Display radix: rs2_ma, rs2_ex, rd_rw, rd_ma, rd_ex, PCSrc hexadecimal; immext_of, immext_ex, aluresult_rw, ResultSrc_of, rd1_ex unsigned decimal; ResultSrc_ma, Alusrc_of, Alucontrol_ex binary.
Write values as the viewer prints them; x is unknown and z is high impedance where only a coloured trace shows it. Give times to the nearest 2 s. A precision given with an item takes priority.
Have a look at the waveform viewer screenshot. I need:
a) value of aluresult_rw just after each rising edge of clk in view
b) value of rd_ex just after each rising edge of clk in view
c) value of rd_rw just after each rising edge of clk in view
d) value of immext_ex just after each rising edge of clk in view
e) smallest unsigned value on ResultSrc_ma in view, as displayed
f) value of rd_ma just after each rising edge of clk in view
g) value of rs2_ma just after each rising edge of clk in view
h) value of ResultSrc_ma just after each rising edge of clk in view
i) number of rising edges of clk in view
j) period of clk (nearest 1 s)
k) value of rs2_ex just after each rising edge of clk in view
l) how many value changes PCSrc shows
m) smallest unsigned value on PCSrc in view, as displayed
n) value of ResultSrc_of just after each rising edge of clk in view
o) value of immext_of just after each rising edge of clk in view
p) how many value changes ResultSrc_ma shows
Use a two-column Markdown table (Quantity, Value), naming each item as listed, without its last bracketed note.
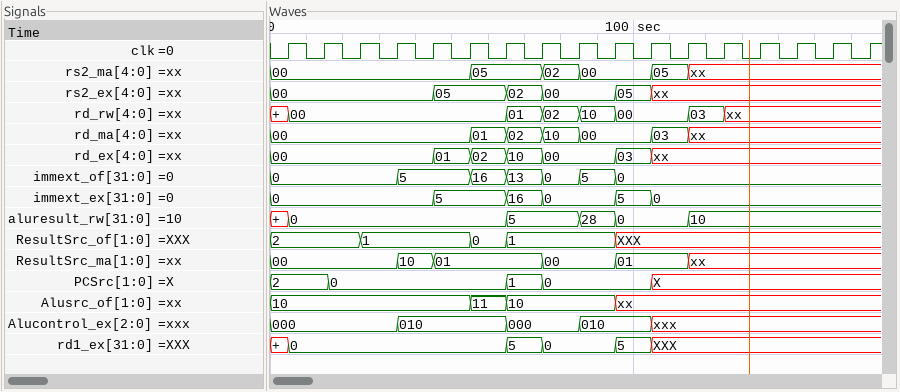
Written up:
| Quantity | Value |
|---|---|
| value of aluresult_rw just after each rising edge of clk in view | 0, 0, 0, 0, 0, 0, 5, 5, 28, 0, 0, 10, 10, 10, 10, 10, 10 |
| value of rd_ex just after each rising edge of clk in view | 00, 00, 00, 00, 01, 02, 10, 00, 00, 03, xx, xx, xx, xx, xx, xx, xx |
| value of rd_rw just after each rising edge of clk in view | 00, 00, 00, 00, 00, 00, 01, 02, 10, 00, 00, 03, xx, xx, xx, xx, xx |
| value of immext_ex just after each rising edge of clk in view | 0, 0, 0, 0, 5, 5, 16, 0, 0, 5, 0, 0, 0, 0, 0, 0, 0 |
| smallest unsigned value on ResultSrc_ma in view, as displayed | 00 |
| value of rd_ma just after each rising edge of clk in view | 00, 00, 00, 00, 00, 01, 02, 10, 00, 00, 03, xx, xx, xx, xx, xx, xx |
| value of rs2_ma just after each rising edge of clk in view | 00, 00, 00, 00, 00, 05, 05, 02, 00, 00, 05, xx, xx, xx, xx, xx, xx |
| value of ResultSrc_ma just after each rising edge of clk in view | 00, 00, 00, 10, 01, 01, 01, 00, 00, 01, 01, xx, xx, xx, xx, xx, xx |
| number of rising edges of clk in view | 17 |
| period of clk | 10 s |
| value of rs2_ex just after each rising edge of clk in view | 00, 00, 00, 00, 05, 05, 02, 00, 00, 05, xx, xx, xx, xx, xx, xx, xx |
| how many value changes PCSrc shows | 4 |
| smallest unsigned value on PCSrc in view, as displayed | 0 |
| value of ResultSrc_of just after each rising edge of clk in view | 2, 2, 1, 1, 1, 0, 1, 1, 1, XXX, XXX, XXX, XXX, XXX, XXX, XXX, XXX |
| value of immext_of just after each rising edge of clk in view | 0, 0, 0, 5, 5, 16, 13, 0, 5, 0, 0, 0, 0, 0, 0, 0, 0 |
| how many value changes ResultSrc_ma shows | 5 |
